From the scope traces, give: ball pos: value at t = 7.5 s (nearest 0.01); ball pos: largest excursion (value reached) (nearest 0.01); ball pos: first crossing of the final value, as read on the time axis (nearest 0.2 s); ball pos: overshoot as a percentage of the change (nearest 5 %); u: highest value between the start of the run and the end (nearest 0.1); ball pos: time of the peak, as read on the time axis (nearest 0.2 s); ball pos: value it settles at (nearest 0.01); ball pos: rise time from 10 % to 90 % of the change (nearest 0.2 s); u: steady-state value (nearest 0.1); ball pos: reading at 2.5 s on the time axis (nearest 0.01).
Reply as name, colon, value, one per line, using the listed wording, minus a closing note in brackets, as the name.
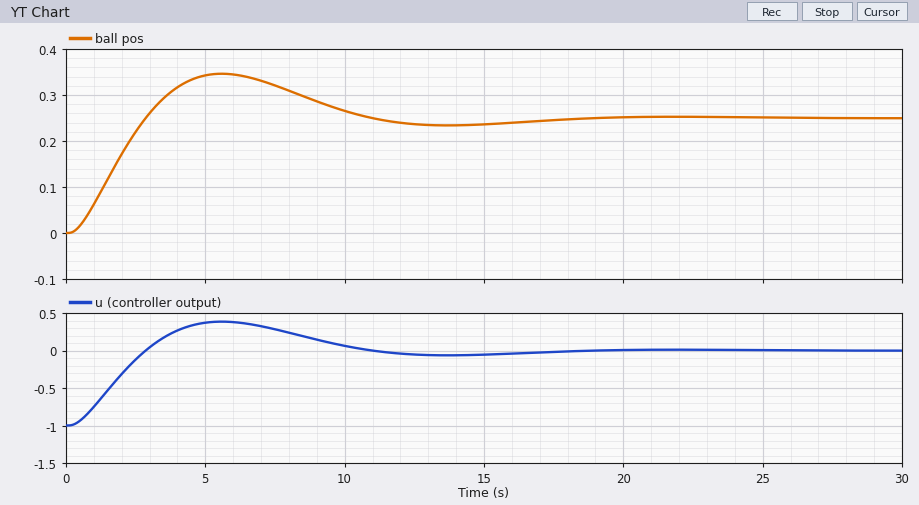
ball pos: value at t = 7.5 s: 0.32
ball pos: largest excursion (value reached): 0.35
ball pos: first crossing of the final value, as read on the time axis: 2.8 s
ball pos: overshoot as a percentage of the change: 40 %
u: highest value between the start of the run and the end: 0.4
ball pos: time of the peak, as read on the time axis: 5.6 s
ball pos: value it settles at: 0.25
ball pos: rise time from 10 % to 90 % of the change: 2.0 s
u: steady-state value: 0.0
ball pos: reading at 2.5 s on the time axis: 0.22
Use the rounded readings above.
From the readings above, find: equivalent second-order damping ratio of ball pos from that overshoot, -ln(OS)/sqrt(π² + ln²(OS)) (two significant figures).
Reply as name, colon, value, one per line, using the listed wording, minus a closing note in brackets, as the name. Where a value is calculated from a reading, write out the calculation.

equivalent second-order damping ratio of ball pos from that overshoot, -ln(OS)/sqrt(π² + ln²(OS)): ln(0.4) = -0.916; 0.916 / sqrt(9.870 + 0.840) = 0.28
